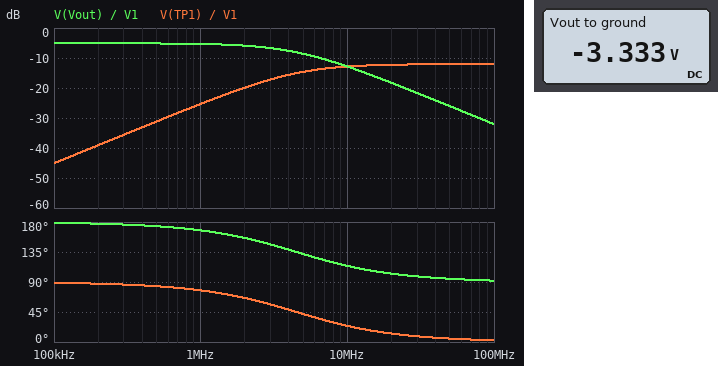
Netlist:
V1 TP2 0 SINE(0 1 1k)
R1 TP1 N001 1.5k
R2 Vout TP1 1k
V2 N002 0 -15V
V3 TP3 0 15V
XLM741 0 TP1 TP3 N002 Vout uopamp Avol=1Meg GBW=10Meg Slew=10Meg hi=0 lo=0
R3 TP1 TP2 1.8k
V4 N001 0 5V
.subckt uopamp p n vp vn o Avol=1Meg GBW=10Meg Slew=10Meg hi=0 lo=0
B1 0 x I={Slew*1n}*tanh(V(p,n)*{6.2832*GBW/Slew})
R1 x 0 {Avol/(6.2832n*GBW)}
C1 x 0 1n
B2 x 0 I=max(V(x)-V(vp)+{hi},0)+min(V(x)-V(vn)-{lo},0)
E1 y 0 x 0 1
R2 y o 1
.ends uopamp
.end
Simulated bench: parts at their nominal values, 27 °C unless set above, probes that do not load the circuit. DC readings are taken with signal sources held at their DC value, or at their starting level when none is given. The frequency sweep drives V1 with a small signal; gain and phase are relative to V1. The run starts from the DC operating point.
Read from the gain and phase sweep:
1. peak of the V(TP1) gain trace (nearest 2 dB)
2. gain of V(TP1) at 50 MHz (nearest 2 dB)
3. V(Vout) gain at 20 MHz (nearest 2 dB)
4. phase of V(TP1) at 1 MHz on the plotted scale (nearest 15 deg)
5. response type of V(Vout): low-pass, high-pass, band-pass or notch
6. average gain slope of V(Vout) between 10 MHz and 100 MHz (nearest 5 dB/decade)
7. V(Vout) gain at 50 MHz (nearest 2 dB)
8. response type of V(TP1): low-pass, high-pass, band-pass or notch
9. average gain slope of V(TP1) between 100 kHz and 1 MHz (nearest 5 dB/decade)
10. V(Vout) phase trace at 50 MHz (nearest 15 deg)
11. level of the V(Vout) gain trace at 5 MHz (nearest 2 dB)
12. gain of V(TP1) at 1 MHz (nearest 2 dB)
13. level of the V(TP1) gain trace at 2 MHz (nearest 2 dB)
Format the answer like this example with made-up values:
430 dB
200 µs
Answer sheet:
-12 dB
-12 dB
-18 dB
75 deg
low-pass
-20 dB/decade
-26 dB
high-pass
20 dB/decade
90 deg
-8 dB
-26 dB
-20 dB
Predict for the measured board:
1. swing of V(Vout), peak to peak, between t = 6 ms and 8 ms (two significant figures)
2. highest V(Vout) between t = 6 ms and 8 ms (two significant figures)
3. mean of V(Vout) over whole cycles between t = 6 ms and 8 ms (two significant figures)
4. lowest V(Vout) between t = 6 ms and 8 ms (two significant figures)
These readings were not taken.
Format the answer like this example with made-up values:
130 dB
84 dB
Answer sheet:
1.1 V
-2.8 V
-3.3 V
-3.9 V
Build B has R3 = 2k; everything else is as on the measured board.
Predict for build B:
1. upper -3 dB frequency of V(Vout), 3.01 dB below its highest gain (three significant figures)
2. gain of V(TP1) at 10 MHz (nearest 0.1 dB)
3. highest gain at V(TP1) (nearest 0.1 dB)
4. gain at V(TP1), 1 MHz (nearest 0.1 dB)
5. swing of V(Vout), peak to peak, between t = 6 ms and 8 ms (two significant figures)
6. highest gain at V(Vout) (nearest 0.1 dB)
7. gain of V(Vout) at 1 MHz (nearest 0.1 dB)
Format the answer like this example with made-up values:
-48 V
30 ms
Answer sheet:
4.61 MHz
-13.6 dB
-12.7 dB
-26.2 dB
1.0 V
-6.0 dB
-6.2 dB
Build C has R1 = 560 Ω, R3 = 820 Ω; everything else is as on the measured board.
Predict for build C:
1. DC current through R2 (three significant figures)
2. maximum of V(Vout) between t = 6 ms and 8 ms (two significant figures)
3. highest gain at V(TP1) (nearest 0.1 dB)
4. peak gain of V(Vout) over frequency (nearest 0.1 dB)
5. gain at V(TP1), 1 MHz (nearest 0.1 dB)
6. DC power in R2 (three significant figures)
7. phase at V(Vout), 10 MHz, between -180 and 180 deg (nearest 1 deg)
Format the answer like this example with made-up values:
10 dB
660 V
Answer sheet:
8.93 mA
-7.7 V
-10.3 dB
1.7 dB
-18.9 dB
79.7 mW
104 deg
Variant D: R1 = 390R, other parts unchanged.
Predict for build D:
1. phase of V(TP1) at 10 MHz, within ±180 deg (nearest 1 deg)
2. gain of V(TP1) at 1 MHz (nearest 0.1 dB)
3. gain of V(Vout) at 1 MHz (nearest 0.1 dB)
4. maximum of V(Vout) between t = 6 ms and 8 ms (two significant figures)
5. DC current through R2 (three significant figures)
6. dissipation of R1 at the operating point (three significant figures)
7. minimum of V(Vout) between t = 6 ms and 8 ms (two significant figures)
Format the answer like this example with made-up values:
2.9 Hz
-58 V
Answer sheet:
14 deg
-25.8 dB
-5.8 dB
-12 V
12.8 mA
64.1 mW
-13 V
